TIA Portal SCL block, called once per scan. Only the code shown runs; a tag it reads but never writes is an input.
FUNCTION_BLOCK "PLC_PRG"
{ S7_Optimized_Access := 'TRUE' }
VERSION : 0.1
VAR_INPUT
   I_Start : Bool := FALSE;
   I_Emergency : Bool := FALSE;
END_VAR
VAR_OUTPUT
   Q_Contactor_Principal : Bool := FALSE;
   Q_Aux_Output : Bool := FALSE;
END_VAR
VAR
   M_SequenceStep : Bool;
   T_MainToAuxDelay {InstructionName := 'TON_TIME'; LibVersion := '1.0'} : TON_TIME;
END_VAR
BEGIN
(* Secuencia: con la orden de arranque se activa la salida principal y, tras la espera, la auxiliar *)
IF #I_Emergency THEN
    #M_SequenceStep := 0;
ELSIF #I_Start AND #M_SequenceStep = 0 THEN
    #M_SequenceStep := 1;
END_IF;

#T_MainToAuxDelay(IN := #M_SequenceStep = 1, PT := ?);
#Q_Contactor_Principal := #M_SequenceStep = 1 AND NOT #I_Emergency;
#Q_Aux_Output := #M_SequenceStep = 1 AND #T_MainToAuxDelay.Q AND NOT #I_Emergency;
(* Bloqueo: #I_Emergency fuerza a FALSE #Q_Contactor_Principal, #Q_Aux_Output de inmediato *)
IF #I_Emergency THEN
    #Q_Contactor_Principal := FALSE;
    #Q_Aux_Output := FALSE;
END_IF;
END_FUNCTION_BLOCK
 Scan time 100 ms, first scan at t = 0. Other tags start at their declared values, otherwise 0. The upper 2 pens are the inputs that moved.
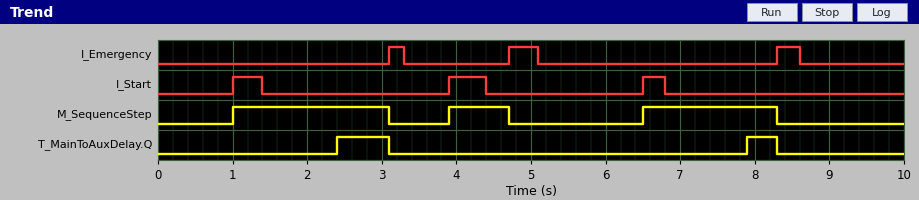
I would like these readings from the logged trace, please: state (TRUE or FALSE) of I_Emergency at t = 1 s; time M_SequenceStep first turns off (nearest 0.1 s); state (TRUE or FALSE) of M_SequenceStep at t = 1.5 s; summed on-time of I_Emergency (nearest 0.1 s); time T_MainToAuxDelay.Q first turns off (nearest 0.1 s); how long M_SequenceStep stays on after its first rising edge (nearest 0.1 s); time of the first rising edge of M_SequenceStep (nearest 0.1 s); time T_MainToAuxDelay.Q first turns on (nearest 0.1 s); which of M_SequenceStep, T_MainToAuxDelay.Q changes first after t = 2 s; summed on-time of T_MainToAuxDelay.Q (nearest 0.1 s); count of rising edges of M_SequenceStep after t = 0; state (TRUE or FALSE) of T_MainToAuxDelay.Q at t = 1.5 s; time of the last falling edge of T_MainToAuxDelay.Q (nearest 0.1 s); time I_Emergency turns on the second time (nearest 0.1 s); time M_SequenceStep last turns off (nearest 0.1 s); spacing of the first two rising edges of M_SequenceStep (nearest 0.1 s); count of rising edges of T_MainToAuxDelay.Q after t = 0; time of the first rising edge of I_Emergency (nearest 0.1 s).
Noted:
FALSE
3.1 s
TRUE
0.9 s
3.1 s
2.1 s
1.0 s
2.4 s
T_MainToAuxDelay.Q
1.1 s
3
FALSE
8.3 s
4.7 s
8.3 s
2.9 s
2
3.1 s
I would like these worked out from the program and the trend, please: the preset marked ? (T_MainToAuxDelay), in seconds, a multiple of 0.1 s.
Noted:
1.4 s
